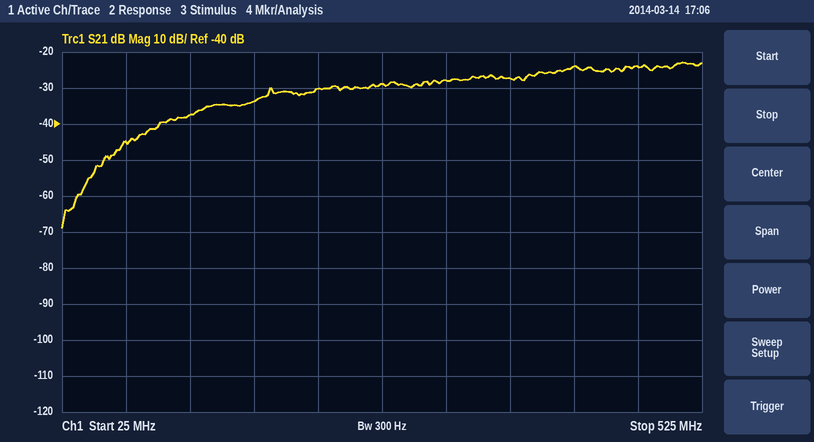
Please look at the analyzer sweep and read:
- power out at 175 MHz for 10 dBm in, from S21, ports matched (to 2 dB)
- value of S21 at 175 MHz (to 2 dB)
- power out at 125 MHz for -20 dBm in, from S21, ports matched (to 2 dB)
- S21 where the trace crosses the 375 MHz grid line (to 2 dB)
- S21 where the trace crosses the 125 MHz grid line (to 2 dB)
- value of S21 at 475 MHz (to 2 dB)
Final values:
-24 dBm
-34 dB
-58 dBm
-28 dB
-38 dB
-24 dB
